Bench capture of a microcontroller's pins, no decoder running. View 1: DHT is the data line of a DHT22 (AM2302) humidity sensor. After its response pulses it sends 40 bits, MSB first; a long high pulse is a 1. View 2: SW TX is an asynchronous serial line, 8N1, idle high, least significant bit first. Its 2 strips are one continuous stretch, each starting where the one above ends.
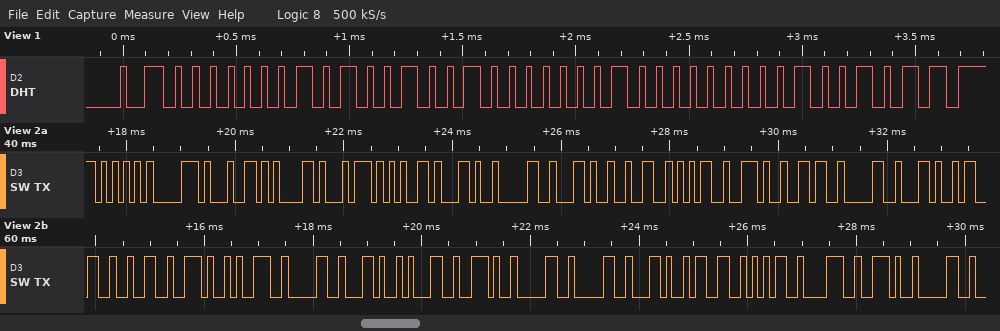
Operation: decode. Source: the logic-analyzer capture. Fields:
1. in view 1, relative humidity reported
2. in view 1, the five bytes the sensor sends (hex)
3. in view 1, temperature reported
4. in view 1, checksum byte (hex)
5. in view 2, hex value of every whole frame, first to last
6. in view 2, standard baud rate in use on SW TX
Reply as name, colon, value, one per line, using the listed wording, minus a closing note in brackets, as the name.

in view 1, relative humidity reported: 32.9 %
in view 1, the five bytes the sensor sends: 01 49 01 00 4B
in view 1, temperature reported: 25.6 °C
in view 1, checksum byte: 0x4B
in view 2, hex value of every whole frame, first to last: 0x55 0x70 0x64 0x61 0x74 0x65 0x2C 0x30 0x2C 0x32 0x35 0x2E 0x36 0x30 0x2C 0x33 0x32 0x2E 0x39 0x30 0x2C 0x31 0x2E 0x30 0x30 0x2C 0x33 0x35 0x38 0x2E 0x30
in view 2, standard baud rate in use on SW TX: 9600 baud
